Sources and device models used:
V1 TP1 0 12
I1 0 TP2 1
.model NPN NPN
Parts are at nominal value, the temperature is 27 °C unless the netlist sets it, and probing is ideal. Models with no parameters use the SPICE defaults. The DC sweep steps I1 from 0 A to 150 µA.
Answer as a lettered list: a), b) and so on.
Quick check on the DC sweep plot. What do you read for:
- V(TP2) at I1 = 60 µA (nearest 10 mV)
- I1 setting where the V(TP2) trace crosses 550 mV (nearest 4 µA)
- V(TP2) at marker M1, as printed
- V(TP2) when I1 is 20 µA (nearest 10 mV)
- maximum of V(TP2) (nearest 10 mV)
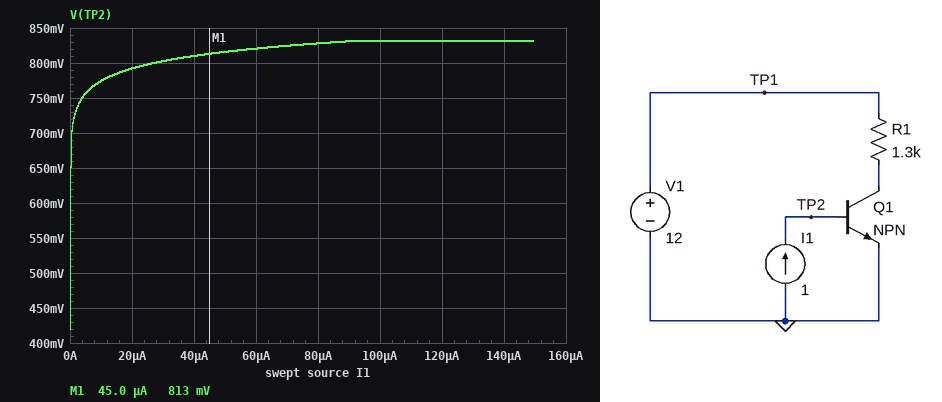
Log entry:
a) 820 mV
b) 0 A
c) 813 mV
d) 790 mV
e) 830 mV
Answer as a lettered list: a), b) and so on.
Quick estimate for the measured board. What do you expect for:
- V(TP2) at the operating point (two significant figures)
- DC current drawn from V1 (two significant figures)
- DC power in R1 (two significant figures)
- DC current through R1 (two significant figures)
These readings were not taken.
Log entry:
a) 970 mV
b) 9.2 mA
c) 110 mW
d) 9.2 mA
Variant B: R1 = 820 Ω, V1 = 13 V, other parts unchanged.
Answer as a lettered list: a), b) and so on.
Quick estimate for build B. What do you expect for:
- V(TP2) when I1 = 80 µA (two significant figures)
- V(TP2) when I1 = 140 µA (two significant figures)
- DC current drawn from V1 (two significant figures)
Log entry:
a) 830 mV
b) 840 mV
c) 16 mA
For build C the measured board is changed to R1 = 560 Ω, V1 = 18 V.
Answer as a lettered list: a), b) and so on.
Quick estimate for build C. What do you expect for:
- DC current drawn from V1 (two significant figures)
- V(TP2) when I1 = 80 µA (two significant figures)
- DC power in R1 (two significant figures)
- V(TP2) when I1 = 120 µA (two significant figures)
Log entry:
a) 32 mA
b) 830 mV
c) 580 mW
d) 840 mV
